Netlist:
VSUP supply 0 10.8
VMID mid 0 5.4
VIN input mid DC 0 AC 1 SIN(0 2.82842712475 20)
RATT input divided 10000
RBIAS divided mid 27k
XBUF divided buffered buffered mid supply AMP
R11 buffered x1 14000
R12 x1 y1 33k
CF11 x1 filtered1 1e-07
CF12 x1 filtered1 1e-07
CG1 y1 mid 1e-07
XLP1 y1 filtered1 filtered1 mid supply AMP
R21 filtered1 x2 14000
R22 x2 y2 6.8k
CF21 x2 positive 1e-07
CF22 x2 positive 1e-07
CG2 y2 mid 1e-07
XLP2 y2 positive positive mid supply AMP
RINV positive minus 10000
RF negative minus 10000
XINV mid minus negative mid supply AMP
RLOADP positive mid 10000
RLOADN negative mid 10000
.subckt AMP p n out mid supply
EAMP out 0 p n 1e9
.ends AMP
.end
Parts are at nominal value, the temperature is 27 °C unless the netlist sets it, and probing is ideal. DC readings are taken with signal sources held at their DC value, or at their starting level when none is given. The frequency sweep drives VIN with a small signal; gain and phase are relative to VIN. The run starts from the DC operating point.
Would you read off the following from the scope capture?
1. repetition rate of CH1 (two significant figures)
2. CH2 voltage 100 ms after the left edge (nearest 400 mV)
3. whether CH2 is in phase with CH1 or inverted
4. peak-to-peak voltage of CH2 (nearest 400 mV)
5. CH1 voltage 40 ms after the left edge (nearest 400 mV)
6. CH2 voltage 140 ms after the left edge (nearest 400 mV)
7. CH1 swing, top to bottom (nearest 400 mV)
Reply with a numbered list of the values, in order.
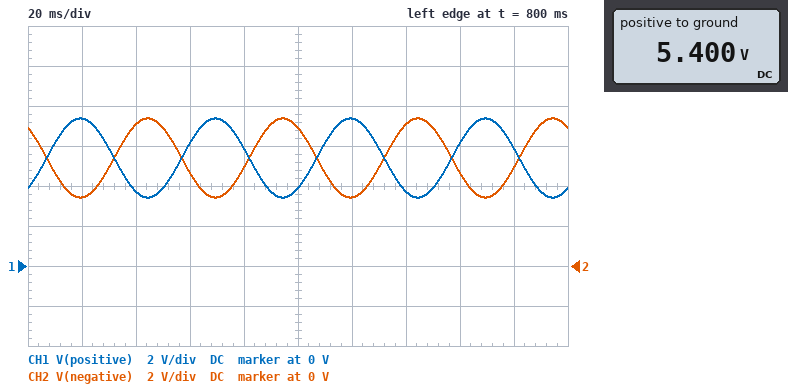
1. 20 Hz
2. 6.8 V
3. inverted
4. 4.0 V
5. 3.6 V
6. 7.2 V
7. 4.0 V
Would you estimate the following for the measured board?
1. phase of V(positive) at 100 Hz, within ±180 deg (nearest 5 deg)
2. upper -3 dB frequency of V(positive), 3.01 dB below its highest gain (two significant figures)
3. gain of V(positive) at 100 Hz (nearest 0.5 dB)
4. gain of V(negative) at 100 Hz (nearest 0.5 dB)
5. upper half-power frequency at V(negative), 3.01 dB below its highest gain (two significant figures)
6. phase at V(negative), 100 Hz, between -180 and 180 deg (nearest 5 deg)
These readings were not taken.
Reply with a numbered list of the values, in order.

1. 150 deg
2. 46 Hz
3. -17.0 dB
4. -17.0 dB
5. 46 Hz
6. -30 deg
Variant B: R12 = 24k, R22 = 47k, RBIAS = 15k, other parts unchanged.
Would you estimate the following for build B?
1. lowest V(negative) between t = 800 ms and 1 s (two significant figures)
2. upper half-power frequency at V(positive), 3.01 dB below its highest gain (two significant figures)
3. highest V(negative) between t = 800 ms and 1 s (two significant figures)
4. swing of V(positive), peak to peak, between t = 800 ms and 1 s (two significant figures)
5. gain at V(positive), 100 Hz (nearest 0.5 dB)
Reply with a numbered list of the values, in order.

1. 3.9 V
2. 33 Hz
3. 6.9 V
4. 3.0 V
5. -29.0 dB
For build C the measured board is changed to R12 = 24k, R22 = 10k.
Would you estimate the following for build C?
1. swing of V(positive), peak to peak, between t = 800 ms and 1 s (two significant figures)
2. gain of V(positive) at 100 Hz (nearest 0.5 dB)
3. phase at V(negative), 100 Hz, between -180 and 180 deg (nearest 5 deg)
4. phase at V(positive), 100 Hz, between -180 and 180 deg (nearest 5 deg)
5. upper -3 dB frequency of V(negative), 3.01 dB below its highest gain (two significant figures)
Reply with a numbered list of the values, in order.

1. 4.1 V
2. -15.5 dB
3. -40 deg
4. 140 deg
5. 55 Hz
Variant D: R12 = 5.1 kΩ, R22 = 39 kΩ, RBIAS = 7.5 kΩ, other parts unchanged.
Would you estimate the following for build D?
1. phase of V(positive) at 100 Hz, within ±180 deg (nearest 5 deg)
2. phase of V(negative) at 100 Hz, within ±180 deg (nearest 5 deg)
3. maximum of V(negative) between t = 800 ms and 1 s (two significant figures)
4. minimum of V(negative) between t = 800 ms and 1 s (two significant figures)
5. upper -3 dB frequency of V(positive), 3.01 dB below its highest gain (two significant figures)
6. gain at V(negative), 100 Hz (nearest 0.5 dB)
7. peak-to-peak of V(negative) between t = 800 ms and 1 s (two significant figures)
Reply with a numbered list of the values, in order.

1. 155 deg
2. -25 deg
3. 6.5 V
4. 4.3 V
5. 40 Hz
6. -23.0 dB
7. 2.3 V
